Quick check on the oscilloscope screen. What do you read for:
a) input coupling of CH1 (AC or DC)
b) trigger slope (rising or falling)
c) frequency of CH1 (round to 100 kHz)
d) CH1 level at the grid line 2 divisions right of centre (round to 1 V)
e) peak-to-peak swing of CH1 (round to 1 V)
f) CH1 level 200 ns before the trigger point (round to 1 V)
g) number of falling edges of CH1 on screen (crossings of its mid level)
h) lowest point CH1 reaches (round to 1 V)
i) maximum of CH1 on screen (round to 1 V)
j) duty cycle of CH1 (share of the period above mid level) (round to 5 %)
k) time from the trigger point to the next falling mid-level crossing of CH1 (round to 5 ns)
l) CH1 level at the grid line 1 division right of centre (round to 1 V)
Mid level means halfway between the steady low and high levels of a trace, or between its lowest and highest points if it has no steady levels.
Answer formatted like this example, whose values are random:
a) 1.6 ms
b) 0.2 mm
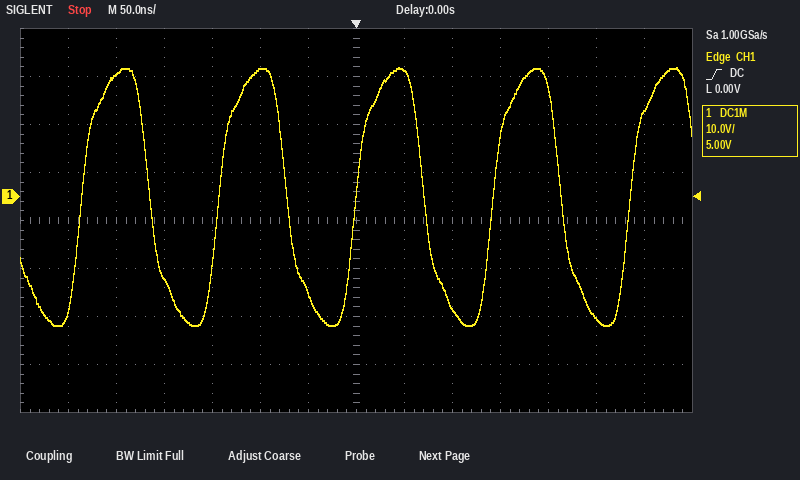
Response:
a) DC
b) rising
c) 7.0 MHz
d) -23 V
e) 54 V
f) -17 V
g) 4
h) -27 V
i) 27 V
j) 50 %
k) 70 ns
l) 26 V
